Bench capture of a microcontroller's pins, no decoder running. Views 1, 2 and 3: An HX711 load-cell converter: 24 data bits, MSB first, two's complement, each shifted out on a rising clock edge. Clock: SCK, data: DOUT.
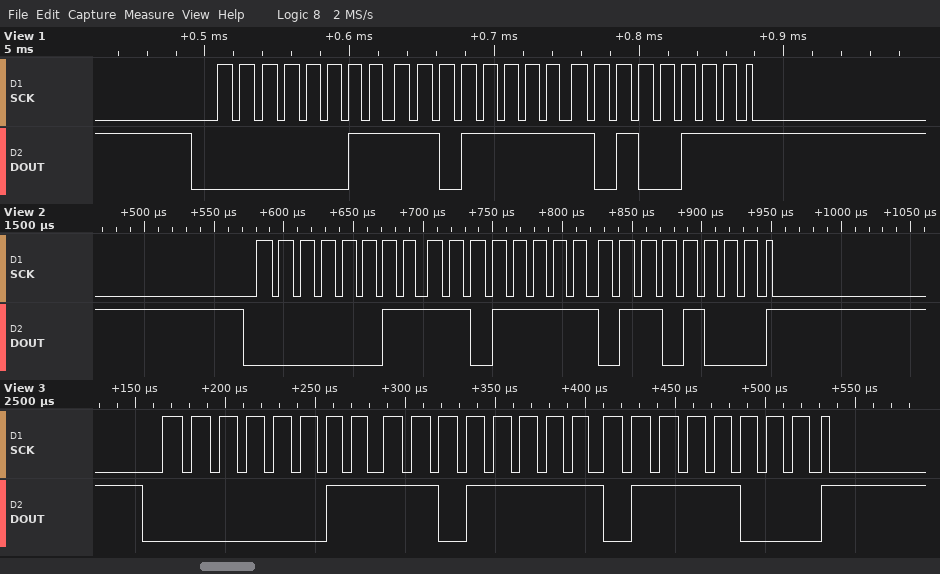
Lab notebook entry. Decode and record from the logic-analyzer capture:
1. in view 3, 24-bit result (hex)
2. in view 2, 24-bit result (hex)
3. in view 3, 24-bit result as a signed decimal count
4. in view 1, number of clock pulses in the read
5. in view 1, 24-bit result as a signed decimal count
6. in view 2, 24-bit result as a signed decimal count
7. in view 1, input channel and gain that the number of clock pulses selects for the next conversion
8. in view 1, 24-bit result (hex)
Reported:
0x03DF78
0x03DF68
253816
25
253863
253800
channel A, gain 128
0x03DFA7
